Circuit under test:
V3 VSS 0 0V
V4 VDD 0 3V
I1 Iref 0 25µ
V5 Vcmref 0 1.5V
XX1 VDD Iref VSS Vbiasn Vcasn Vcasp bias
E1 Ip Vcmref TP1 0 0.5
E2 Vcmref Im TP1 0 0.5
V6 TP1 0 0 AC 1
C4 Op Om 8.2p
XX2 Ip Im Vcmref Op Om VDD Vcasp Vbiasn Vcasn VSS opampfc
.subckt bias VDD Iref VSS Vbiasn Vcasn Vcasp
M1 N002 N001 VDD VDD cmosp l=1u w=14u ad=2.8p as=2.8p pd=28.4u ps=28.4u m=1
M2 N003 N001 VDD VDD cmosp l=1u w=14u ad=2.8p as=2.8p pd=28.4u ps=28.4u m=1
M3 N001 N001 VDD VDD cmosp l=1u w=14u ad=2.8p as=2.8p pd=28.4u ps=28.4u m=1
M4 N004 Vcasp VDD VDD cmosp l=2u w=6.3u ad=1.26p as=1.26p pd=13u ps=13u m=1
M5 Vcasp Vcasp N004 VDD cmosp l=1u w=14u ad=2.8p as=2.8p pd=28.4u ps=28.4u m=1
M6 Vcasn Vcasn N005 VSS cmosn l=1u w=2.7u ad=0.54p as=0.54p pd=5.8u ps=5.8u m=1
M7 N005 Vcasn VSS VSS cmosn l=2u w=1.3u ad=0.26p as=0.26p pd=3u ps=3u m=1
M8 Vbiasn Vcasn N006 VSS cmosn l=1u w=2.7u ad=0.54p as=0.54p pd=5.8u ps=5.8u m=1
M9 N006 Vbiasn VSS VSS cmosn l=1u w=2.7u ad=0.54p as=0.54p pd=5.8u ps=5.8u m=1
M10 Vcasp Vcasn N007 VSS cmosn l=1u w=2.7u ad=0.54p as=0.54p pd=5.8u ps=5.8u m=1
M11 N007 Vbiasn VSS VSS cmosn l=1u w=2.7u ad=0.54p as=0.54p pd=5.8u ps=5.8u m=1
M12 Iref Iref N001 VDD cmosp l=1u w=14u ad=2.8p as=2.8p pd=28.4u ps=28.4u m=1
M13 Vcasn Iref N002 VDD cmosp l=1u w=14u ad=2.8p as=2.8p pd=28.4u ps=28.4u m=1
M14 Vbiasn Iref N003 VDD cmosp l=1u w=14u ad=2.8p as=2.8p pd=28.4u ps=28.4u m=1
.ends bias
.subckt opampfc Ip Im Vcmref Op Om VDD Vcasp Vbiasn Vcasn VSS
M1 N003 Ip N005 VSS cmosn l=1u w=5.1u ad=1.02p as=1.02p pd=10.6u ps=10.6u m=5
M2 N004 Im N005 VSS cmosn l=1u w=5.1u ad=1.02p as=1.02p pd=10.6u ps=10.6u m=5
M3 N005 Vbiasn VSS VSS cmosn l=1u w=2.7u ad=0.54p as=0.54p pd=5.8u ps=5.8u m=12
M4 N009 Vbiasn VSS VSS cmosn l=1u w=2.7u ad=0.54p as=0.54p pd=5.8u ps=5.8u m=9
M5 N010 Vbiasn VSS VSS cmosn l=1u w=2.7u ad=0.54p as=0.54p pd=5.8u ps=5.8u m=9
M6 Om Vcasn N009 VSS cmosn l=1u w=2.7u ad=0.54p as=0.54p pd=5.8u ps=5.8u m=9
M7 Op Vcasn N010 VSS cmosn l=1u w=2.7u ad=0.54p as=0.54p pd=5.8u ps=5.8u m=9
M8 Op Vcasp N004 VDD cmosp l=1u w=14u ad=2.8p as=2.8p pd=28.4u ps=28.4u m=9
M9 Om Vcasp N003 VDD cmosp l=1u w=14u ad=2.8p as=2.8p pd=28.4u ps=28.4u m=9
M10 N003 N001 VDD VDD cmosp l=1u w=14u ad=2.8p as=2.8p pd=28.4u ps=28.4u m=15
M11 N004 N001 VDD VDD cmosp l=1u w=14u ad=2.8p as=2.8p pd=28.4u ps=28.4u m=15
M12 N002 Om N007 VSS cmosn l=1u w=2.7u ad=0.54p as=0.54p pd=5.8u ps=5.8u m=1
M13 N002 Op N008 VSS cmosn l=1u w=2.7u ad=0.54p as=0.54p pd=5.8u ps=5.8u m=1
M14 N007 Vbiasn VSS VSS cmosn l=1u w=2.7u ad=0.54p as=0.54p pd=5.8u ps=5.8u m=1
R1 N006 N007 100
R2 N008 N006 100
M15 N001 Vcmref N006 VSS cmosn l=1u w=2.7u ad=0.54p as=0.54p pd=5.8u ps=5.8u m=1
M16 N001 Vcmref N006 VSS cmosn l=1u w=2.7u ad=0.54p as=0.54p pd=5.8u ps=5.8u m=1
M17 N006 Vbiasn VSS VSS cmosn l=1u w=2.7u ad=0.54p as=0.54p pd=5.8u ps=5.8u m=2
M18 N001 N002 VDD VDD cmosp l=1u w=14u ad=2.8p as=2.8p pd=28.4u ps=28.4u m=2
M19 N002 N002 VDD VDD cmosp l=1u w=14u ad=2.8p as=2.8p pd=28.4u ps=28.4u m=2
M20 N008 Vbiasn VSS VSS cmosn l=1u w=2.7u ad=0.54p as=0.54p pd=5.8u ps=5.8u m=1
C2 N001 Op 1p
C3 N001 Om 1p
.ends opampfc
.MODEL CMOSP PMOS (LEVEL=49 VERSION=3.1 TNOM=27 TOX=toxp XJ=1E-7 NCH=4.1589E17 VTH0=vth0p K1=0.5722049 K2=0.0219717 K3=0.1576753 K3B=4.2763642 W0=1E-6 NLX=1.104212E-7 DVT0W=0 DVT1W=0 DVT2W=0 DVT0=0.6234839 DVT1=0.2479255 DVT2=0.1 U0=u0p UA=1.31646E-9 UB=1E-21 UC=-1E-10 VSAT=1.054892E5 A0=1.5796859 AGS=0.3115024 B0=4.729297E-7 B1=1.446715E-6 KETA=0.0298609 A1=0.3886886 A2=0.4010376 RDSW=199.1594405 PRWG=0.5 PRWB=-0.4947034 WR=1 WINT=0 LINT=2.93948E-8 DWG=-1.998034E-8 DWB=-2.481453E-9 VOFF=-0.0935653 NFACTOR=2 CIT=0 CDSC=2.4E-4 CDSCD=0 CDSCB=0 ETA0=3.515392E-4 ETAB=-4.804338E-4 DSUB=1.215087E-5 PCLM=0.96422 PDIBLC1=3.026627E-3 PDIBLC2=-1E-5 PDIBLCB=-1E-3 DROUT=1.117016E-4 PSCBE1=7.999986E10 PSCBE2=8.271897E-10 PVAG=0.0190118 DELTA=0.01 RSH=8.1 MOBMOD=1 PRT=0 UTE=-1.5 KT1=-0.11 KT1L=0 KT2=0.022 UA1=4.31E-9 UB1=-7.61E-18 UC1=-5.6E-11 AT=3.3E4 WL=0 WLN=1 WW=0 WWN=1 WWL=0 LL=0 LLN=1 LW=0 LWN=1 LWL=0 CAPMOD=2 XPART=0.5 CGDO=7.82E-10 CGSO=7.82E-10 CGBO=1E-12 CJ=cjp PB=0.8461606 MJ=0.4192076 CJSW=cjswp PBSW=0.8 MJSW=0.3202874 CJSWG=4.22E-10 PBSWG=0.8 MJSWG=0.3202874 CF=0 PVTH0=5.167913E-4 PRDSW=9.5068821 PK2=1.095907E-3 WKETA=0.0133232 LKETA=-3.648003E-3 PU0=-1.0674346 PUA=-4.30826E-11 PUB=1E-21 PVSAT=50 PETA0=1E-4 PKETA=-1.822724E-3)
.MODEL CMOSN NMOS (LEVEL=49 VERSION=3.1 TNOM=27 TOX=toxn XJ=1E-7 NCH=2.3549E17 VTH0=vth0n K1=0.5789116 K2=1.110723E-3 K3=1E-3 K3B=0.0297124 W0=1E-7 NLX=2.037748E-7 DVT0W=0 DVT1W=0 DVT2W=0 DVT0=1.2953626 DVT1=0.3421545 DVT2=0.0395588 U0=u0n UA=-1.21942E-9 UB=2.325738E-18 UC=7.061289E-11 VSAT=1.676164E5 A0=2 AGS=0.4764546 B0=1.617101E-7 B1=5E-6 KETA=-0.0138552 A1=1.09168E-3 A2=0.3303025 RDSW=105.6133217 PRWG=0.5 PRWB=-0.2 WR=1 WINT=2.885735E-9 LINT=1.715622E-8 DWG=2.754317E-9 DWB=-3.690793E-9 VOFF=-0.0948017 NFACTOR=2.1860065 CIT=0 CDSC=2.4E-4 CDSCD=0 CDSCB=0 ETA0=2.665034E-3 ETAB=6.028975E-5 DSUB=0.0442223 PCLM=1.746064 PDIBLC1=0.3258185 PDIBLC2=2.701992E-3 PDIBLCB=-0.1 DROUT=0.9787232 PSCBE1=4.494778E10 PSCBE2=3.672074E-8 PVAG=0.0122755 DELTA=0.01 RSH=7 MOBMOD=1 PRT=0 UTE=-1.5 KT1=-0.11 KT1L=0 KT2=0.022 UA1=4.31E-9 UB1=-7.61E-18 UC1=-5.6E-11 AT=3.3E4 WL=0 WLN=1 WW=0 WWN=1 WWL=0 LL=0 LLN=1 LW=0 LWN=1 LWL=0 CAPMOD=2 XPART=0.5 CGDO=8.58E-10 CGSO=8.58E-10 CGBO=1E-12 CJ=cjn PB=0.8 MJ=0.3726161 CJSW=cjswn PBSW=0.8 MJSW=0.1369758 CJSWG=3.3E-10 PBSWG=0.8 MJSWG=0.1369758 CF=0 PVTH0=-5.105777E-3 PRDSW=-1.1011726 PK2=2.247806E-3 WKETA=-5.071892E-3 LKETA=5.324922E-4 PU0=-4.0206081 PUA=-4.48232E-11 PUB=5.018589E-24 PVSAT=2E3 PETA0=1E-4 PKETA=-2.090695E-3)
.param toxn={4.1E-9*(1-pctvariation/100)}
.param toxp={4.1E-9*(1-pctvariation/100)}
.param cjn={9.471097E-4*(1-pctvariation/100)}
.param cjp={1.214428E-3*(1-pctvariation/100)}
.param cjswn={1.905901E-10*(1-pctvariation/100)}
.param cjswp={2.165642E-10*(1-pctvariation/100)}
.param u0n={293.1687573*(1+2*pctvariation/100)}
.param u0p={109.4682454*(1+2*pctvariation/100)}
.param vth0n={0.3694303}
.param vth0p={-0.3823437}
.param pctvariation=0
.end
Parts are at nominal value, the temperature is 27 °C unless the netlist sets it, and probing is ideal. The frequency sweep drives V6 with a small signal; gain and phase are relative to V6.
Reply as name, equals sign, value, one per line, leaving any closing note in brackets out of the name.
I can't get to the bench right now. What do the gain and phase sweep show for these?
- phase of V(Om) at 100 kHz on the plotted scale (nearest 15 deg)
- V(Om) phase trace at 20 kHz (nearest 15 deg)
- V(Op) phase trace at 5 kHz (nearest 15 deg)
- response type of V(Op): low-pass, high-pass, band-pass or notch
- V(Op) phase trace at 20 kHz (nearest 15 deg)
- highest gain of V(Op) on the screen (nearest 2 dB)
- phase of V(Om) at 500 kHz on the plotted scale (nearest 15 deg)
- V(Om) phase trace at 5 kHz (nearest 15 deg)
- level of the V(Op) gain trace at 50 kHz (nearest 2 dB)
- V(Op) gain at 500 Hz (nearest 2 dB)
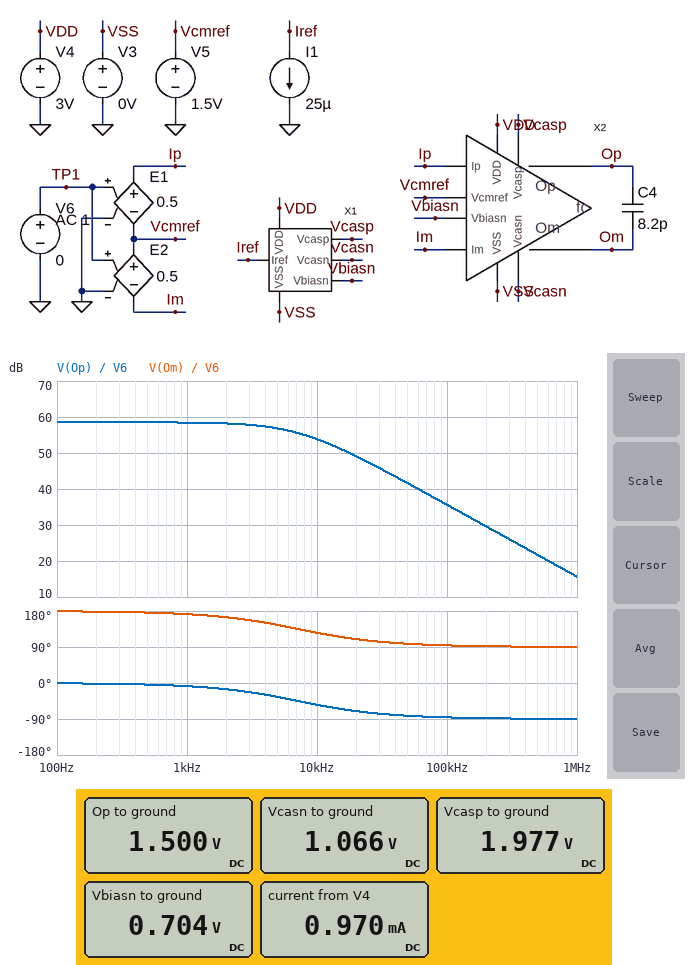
phase of V(Om) at 100 kHz on the plotted scale = 90 deg
V(Om) phase trace at 20 kHz = 105 deg
V(Op) phase trace at 5 kHz = -30 deg
response type of V(Op): low-pass, high-pass, band-pass or notch = low-pass
V(Op) phase trace at 20 kHz = -75 deg
highest gain of V(Op) on the screen = 58 dB
phase of V(Om) at 500 kHz on the plotted scale = 90 deg
V(Om) phase trace at 5 kHz = 150 deg
level of the V(Op) gain trace at 50 kHz = 42 dB
V(Op) gain at 500 Hz = 58 dB
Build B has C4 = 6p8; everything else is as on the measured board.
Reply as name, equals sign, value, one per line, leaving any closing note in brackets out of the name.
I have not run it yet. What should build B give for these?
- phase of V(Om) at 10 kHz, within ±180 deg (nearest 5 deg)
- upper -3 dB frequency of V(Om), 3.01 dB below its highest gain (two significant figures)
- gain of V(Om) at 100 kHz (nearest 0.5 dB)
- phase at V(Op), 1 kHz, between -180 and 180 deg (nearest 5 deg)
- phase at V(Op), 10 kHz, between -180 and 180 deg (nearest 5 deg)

phase of V(Om) at 10 kHz, within ±180 deg = 130 deg
upper -3 dB frequency of V(Om), 3.01 dB below its highest gain = 8.5 kHz
gain of V(Om) at 100 kHz = 37.0 dB
phase at V(Op), 1 kHz, between -180 and 180 deg = -5 deg
phase at V(Op), 10 kHz, between -180 and 180 deg = -50 deg
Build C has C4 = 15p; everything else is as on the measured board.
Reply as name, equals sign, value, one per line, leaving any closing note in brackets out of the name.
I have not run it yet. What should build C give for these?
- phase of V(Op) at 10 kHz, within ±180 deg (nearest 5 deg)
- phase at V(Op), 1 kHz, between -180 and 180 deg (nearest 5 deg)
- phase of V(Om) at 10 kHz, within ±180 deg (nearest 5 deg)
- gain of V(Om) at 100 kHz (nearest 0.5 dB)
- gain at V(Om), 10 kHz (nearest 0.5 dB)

phase of V(Op) at 10 kHz, within ±180 deg = -70 deg
phase at V(Op), 1 kHz, between -180 and 180 deg = -15 deg
phase of V(Om) at 10 kHz, within ±180 deg = 110 deg
gain of V(Om) at 100 kHz = 30.5 dB
gain at V(Om), 10 kHz = 50.0 dB
